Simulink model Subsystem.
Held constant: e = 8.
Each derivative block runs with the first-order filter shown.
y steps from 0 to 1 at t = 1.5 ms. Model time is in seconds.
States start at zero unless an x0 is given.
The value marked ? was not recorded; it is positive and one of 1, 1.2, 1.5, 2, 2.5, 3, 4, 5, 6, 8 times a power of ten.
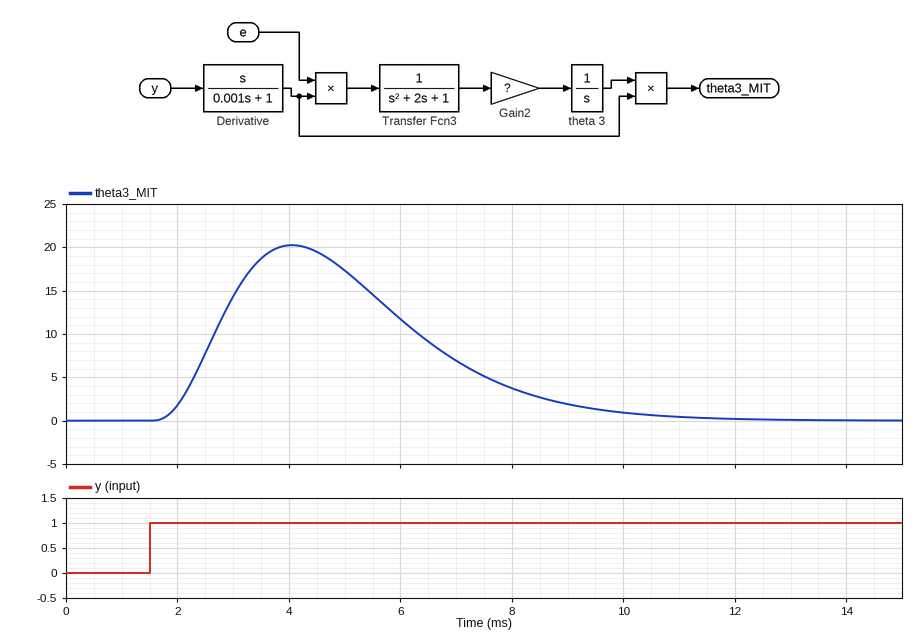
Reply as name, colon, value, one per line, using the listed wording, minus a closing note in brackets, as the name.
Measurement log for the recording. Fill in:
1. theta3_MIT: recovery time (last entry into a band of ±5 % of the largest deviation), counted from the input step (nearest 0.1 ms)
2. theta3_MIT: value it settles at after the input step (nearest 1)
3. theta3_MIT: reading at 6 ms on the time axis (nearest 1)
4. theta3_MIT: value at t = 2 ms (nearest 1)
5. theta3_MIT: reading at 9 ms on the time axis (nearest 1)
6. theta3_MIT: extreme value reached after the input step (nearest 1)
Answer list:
theta3_MIT: recovery time (last entry into a band of ±5 % of the largest deviation), counted from the input step: 8.4 ms
theta3_MIT: value it settles at after the input step: 0
theta3_MIT: reading at 6 ms on the time axis: 12
theta3_MIT: value at t = 2 ms: 2
theta3_MIT: reading at 9 ms on the time axis: 2
theta3_MIT: extreme value reached after the input step: 20
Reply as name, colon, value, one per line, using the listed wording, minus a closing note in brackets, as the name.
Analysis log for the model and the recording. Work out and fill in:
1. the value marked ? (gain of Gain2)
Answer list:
the value marked ?: 20000
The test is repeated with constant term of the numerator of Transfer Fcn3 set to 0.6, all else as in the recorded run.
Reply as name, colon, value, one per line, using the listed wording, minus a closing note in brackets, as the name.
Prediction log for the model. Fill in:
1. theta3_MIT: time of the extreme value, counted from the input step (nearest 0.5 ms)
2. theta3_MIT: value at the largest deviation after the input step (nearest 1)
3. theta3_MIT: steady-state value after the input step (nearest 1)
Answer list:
theta3_MIT: time of the extreme value, counted from the input step: 2.5 ms
theta3_MIT: value at the largest deviation after the input step: 12
theta3_MIT: steady-state value after the input step: 0
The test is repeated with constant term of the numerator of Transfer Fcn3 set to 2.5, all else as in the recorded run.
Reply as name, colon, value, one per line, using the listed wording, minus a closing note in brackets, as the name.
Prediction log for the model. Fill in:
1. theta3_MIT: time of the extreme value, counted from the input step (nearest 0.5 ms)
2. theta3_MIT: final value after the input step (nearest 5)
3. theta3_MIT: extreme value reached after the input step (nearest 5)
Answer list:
theta3_MIT: time of the extreme value, counted from the input step: 2.5 ms
theta3_MIT: final value after the input step: 0
theta3_MIT: extreme value reached after the input step: 50
